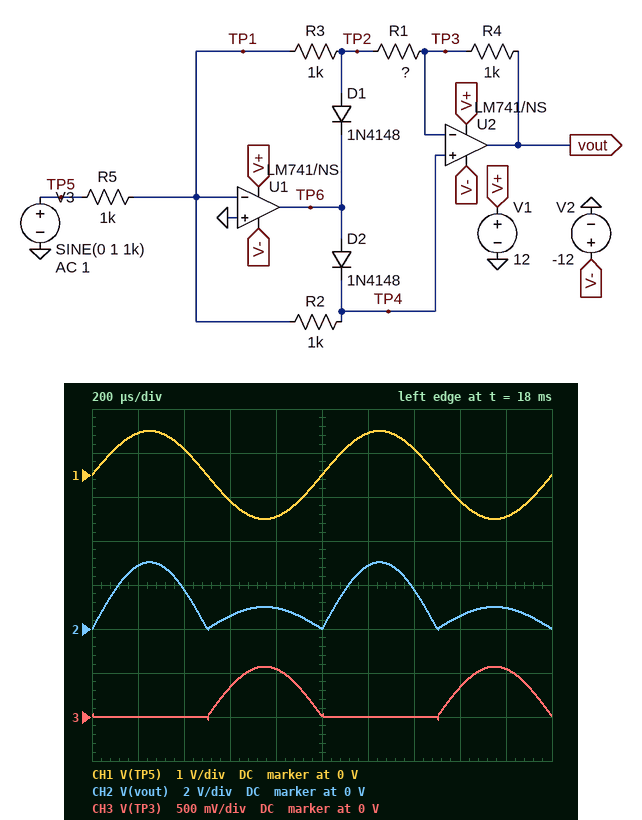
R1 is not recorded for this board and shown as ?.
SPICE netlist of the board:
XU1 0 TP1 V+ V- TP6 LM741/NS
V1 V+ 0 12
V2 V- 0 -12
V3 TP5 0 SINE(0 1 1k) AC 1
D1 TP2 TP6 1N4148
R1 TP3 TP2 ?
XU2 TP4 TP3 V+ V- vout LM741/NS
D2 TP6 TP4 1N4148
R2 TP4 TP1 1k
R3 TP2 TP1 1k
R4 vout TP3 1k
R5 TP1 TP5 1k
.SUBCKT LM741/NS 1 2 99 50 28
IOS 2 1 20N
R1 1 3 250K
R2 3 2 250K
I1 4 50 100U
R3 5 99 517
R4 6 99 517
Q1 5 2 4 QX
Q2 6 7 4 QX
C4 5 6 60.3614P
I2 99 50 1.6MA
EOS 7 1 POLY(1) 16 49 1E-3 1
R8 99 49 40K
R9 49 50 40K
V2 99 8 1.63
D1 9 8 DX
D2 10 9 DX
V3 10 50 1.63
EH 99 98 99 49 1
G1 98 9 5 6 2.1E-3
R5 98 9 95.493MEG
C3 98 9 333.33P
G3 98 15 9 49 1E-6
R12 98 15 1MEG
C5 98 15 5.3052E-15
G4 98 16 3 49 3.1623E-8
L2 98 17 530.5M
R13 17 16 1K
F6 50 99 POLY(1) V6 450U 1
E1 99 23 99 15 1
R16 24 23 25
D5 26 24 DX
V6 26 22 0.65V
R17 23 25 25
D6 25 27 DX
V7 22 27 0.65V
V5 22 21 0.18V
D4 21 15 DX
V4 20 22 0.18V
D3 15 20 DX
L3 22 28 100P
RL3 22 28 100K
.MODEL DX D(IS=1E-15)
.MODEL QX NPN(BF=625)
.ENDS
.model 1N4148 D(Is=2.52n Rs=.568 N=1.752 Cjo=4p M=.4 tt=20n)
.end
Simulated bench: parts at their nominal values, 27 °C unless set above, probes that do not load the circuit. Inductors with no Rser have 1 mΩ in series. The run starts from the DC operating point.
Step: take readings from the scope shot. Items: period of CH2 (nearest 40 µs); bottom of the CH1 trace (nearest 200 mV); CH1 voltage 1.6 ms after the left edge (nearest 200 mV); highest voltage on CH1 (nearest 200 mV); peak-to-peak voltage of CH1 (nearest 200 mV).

1.00 ms
-1.0 V
-600 mV
1.0 V
2.0 V
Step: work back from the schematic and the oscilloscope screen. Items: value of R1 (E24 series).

330 Ω
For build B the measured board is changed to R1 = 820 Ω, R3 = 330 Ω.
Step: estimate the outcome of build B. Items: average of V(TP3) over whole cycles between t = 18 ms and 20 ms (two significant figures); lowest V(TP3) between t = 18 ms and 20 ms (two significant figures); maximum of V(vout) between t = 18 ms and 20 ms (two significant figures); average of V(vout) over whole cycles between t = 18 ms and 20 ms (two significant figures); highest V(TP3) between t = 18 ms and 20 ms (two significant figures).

170 mV
-30 mV
1.0 V
450 mV
540 mV
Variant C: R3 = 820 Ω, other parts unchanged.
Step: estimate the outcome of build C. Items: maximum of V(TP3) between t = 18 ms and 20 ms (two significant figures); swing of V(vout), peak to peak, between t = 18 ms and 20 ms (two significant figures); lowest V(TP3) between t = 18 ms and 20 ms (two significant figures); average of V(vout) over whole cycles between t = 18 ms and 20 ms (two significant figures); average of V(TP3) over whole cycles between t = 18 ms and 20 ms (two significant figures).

540 mV
2.5 V
-32 mV
1.1 V
170 mV
